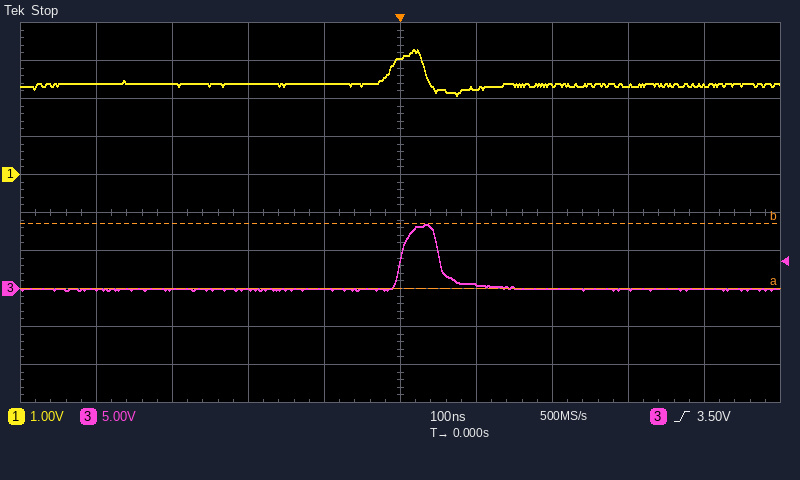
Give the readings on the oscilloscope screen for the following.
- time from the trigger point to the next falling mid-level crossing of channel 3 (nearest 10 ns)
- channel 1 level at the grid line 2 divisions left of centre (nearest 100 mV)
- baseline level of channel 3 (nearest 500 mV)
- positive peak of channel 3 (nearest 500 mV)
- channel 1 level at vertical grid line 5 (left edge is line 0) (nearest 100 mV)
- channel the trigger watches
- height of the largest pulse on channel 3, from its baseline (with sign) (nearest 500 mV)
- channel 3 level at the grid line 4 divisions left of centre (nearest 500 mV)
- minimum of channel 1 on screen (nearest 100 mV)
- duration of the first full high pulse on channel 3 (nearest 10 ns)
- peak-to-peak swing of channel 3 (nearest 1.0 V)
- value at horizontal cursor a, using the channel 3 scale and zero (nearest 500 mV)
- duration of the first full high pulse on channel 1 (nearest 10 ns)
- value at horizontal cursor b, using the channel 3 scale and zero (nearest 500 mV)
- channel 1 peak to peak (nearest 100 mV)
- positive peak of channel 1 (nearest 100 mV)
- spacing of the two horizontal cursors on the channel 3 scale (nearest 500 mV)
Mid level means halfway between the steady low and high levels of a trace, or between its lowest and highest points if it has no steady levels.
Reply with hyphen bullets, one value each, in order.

- 50 ns
- 2.4 V
- 0.0 V
- 8.5 V
- 3.1 V
- channel 3
- +8.5 V
- 0.0 V
- 2.1 V
- 50 ns
- 9.0 V
- 0.0 V
- 50 ns
- 8.5 V
- 1.2 V
- 3.3 V
- 8.5 V
